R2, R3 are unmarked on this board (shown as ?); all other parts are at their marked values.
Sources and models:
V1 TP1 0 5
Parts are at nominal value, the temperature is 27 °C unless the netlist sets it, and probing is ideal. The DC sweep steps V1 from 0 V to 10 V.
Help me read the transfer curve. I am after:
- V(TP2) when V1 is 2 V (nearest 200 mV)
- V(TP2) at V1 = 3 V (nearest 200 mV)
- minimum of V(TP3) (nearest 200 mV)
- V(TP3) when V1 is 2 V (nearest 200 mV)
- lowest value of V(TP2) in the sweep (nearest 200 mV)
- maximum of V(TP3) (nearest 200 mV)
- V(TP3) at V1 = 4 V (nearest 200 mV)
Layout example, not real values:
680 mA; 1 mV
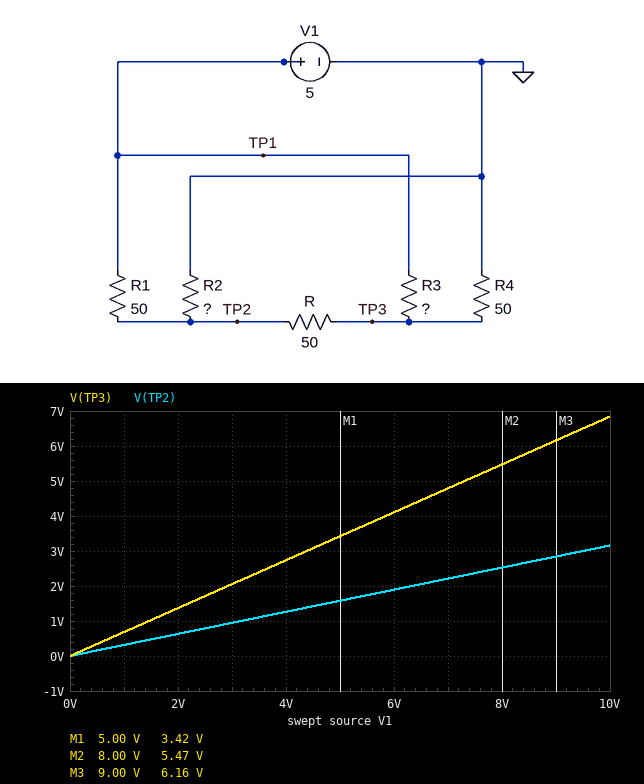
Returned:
600 mV; 1.0 V; 0 V; 1.4 V; 0 V; 6.8 V; 2.8 V
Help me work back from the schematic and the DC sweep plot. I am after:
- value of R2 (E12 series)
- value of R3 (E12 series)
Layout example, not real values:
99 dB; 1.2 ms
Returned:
15 Ω; 15 Ω
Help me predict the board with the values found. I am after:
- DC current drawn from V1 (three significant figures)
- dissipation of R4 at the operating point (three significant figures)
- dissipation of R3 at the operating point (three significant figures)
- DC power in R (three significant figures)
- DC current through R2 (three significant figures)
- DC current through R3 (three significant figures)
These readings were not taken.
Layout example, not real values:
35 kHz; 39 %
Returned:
174 mA; 234 mW; 166 mW; 67.9 mW; 105 mA; 105 mA
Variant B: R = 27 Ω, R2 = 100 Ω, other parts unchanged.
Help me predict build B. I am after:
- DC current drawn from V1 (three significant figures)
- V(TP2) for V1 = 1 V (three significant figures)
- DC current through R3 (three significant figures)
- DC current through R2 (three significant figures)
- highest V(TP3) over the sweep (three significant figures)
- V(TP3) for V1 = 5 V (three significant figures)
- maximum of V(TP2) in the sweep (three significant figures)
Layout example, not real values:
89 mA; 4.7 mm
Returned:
111 mA; 714 mV; 82.4 mA; 35.7 mA; 7.53 V; 3.76 V; 7.14 V
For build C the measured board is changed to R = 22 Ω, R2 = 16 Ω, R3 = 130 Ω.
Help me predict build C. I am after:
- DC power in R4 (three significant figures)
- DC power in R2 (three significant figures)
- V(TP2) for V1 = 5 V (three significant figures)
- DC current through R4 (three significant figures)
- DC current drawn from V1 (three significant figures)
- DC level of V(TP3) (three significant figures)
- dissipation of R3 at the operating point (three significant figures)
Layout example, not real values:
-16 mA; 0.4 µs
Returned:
33.7 mW; 96.5 mW; 1.24 V; 26.0 mA; 104 mA; 1.30 V; 105 mW
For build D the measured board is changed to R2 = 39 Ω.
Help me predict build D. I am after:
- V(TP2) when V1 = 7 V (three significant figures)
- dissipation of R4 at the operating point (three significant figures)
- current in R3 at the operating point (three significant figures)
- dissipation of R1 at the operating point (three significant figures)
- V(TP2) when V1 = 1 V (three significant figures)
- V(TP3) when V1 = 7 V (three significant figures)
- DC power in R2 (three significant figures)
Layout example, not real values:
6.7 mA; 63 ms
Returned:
3.68 V; 262 mW; 92.2 mA; 113 mW; 525 mV; 5.06 V; 177 mW
